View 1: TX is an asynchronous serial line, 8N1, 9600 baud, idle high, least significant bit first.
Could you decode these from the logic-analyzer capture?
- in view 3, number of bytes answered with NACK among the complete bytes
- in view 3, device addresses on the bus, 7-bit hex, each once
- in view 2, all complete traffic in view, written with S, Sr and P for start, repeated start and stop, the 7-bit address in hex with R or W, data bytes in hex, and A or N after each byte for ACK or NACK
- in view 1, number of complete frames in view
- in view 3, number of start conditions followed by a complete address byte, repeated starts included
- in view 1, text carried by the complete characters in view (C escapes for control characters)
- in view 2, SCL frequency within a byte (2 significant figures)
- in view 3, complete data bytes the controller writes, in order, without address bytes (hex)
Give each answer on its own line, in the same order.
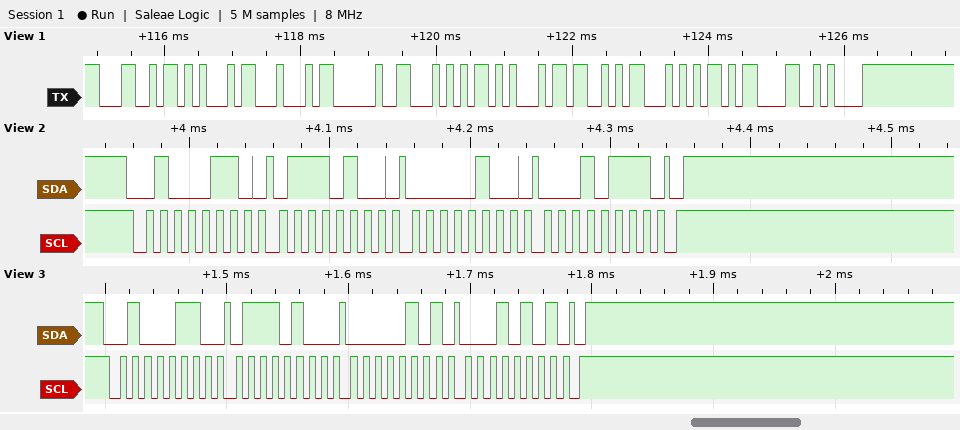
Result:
0
0x23
S 23W A 74 A 04 A 17 A P
10
1
"LED TEST\r\n"
100 kHz
74 05 15
